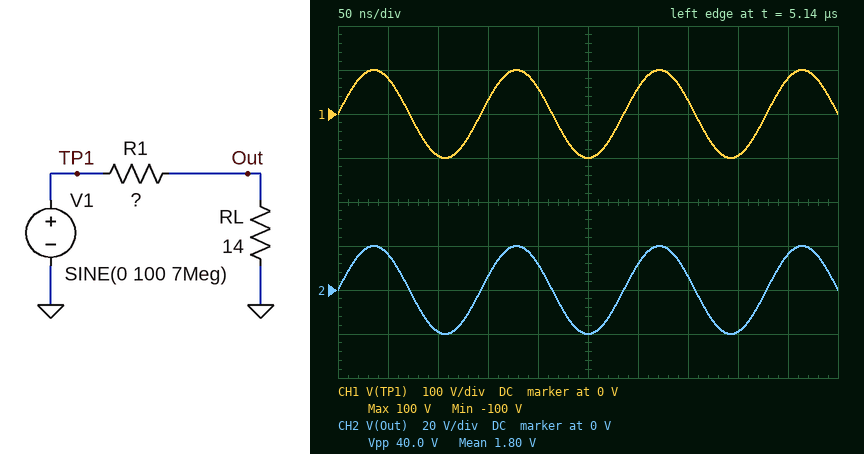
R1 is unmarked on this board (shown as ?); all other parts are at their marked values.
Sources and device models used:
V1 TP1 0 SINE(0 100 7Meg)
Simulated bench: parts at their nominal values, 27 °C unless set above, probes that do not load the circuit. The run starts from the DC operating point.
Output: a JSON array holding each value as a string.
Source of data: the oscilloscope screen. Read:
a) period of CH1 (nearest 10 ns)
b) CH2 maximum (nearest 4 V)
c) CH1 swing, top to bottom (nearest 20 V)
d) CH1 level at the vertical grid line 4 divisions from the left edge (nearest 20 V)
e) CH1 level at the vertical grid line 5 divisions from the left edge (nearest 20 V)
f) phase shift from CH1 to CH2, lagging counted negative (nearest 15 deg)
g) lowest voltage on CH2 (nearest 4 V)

["140 ns", "20 V", "200 V", "60 V", "-100 V", "0 deg", "-20 V"]
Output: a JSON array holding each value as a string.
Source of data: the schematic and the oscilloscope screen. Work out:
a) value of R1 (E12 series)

["56 Ω"]
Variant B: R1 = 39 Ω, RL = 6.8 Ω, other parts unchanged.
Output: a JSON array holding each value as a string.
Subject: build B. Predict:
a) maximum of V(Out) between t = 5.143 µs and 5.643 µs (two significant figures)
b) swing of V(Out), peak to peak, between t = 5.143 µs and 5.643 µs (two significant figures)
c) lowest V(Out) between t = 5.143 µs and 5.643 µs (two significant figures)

["15 V", "30 V", "-15 V"]
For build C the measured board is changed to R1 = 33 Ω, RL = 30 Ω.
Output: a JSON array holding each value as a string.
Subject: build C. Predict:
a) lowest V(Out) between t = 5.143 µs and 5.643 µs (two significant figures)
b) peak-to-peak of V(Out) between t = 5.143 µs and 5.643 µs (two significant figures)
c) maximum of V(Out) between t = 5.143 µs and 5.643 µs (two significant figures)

["-48 V", "95 V", "48 V"]
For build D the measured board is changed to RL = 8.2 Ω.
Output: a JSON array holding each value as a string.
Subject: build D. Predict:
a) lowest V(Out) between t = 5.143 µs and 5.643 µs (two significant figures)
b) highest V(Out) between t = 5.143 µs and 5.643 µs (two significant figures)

["-13 V", "13 V"]
